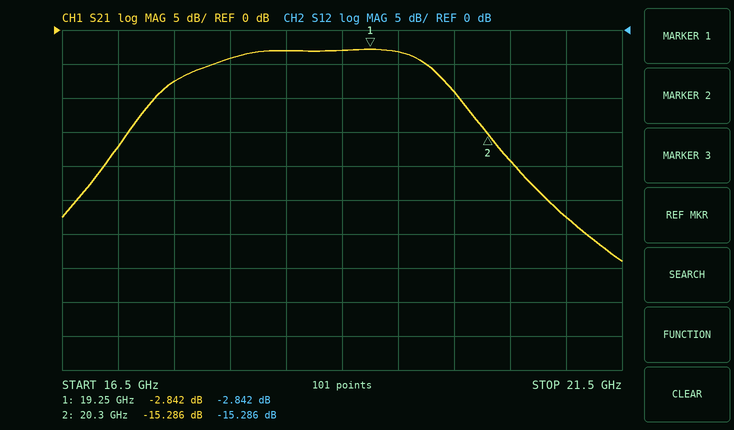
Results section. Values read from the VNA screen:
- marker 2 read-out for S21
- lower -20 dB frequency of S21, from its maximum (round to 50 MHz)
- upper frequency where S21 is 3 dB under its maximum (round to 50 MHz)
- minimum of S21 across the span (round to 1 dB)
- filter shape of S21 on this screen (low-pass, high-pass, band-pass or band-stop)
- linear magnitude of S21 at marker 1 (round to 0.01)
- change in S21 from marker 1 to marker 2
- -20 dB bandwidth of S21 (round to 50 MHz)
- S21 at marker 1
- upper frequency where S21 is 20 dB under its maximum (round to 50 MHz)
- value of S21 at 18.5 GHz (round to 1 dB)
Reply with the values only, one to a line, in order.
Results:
-15.286 dB
16.75 GHz
19.80 GHz
-34 dB
band-pass
0.72
-12.444 dB
3.95 GHz
-2.842 dB
20.70 GHz
-3 dB
